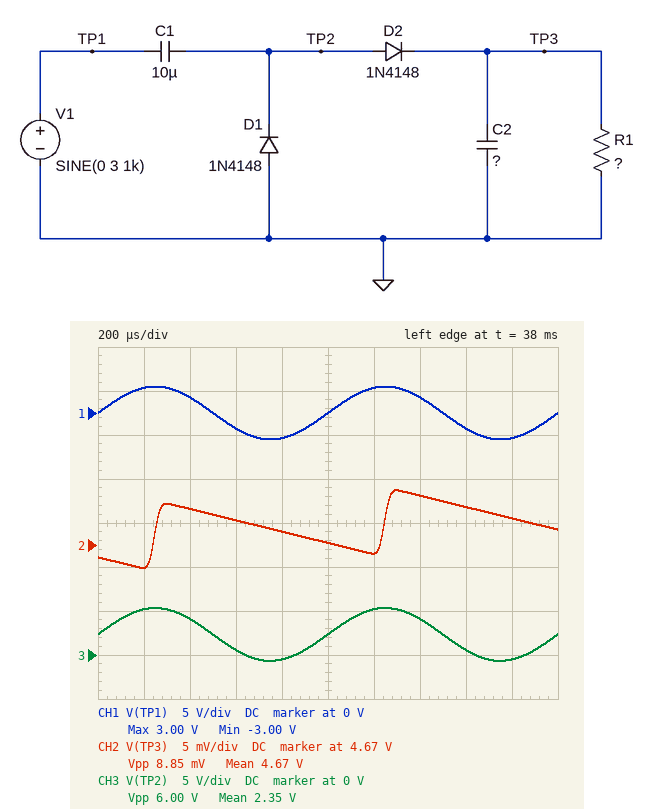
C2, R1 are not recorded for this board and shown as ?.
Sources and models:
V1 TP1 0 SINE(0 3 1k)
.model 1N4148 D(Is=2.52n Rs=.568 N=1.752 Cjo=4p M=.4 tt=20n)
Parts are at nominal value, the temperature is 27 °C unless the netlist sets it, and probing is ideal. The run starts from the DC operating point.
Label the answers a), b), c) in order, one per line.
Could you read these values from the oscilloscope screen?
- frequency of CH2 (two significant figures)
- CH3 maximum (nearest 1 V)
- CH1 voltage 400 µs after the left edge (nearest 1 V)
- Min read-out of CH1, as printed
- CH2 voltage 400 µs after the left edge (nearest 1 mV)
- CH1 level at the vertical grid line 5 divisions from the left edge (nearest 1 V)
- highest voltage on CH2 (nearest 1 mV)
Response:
a) 1.0 kHz
b) 5 V
c) 2 V
d) -3.00 V
e) 4.674 V
f) 0 V
g) 4.676 V
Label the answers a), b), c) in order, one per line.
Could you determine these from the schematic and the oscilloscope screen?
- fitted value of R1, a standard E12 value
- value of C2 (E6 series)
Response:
a) 22 kΩ
b) 33 µF
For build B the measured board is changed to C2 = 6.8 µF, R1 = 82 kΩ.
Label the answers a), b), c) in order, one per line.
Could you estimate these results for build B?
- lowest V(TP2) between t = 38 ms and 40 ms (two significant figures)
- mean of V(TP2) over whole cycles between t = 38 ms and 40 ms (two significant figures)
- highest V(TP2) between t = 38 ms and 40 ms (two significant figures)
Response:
a) -600 mV
b) 2.4 V
c) 5.4 V
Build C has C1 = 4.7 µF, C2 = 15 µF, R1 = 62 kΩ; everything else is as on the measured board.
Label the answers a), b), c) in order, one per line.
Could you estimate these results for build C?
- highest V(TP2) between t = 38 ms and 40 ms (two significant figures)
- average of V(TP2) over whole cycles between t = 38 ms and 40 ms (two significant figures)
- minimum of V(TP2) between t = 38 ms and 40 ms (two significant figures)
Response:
a) 5.4 V
b) 2.4 V
c) -620 mV
